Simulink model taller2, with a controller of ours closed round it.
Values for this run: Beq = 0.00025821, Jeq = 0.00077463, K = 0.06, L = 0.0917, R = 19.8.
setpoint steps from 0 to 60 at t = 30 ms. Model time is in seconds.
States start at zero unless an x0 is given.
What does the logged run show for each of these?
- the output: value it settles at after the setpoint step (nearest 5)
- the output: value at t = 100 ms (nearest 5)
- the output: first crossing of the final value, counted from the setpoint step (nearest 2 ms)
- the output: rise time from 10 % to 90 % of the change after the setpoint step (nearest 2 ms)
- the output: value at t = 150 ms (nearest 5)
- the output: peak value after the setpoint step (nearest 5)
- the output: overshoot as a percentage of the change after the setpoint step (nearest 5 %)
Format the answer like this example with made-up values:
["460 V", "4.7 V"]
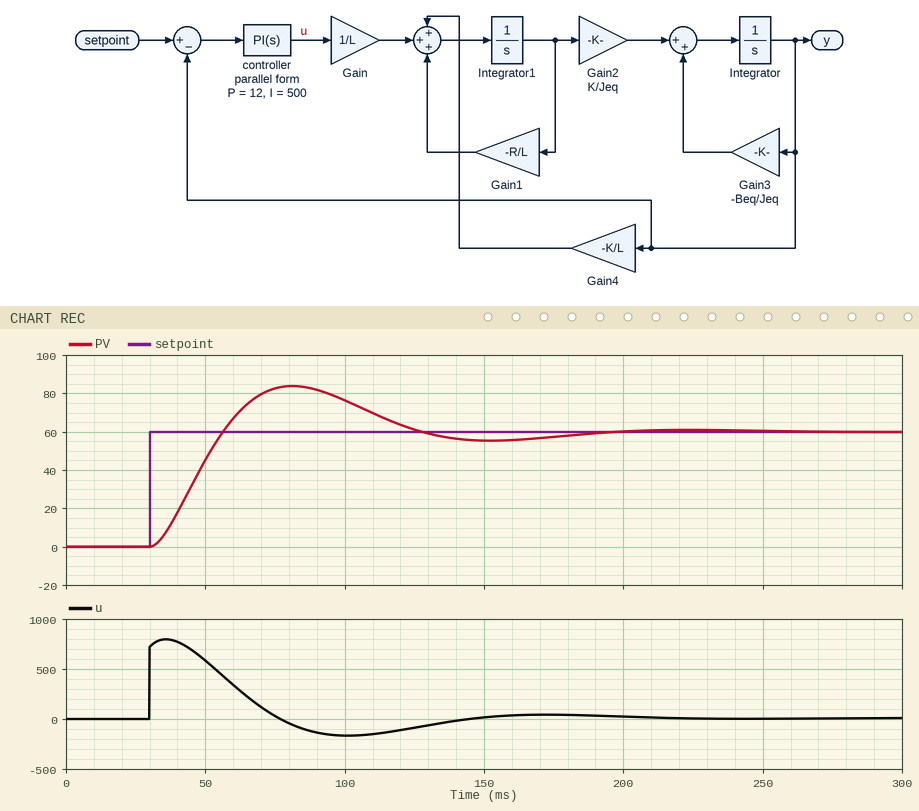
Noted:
["60", "75", "26 ms", "18 ms", "55", "85", "40 %"]
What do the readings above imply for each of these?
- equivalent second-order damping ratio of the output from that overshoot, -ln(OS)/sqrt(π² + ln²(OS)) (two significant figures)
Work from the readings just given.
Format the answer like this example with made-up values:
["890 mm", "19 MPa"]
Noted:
["0.28"]
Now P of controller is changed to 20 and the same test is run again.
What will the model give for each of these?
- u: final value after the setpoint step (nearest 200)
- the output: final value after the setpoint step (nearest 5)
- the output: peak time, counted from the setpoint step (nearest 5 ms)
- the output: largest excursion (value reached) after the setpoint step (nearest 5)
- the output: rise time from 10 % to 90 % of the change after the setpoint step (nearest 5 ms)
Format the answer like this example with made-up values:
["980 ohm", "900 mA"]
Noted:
["0", "60", "40 ms", "75", "15 ms"]
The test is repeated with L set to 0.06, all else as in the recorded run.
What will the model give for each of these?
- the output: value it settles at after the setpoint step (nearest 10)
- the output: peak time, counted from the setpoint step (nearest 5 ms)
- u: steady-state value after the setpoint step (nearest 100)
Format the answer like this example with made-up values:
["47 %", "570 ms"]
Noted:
["60", "50 ms", "0"]
